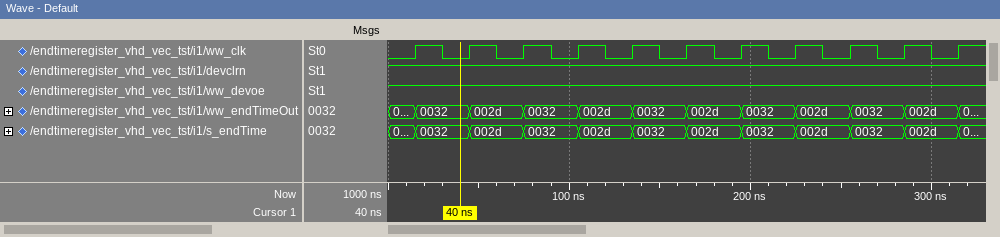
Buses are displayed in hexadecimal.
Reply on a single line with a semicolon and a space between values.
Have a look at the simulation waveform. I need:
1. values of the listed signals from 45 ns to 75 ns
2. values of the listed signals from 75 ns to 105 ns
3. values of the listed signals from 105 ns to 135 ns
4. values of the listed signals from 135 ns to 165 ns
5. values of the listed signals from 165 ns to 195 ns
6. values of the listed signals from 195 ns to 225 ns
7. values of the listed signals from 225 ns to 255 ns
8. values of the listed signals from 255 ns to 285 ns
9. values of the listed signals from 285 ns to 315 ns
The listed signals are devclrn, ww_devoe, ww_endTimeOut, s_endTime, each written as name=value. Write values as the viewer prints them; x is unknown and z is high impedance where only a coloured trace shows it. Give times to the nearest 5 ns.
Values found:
devclrn=1, ww_devoe=1, ww_endTimeOut=002d, s_endTime=002d; devclrn=1, ww_devoe=1, ww_endTimeOut=0032, s_endTime=0032; devclrn=1, ww_devoe=1, ww_endTimeOut=002d, s_endTime=002d; devclrn=1, ww_devoe=1, ww_endTimeOut=0032, s_endTime=0032; devclrn=1, ww_devoe=1, ww_endTimeOut=002d, s_endTime=002d; devclrn=1, ww_devoe=1, ww_endTimeOut=0032, s_endTime=0032; devclrn=1, ww_devoe=1, ww_endTimeOut=002d, s_endTime=002d; devclrn=1, ww_devoe=1, ww_endTimeOut=0032, s_endTime=0032; devclrn=1, ww_devoe=1, ww_endTimeOut=002d, s_endTime=002d
